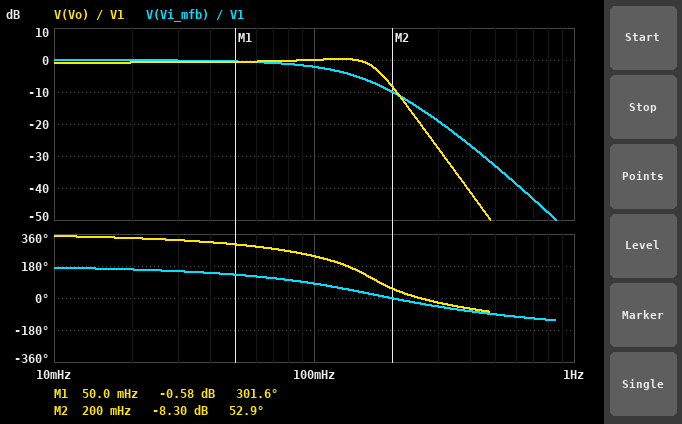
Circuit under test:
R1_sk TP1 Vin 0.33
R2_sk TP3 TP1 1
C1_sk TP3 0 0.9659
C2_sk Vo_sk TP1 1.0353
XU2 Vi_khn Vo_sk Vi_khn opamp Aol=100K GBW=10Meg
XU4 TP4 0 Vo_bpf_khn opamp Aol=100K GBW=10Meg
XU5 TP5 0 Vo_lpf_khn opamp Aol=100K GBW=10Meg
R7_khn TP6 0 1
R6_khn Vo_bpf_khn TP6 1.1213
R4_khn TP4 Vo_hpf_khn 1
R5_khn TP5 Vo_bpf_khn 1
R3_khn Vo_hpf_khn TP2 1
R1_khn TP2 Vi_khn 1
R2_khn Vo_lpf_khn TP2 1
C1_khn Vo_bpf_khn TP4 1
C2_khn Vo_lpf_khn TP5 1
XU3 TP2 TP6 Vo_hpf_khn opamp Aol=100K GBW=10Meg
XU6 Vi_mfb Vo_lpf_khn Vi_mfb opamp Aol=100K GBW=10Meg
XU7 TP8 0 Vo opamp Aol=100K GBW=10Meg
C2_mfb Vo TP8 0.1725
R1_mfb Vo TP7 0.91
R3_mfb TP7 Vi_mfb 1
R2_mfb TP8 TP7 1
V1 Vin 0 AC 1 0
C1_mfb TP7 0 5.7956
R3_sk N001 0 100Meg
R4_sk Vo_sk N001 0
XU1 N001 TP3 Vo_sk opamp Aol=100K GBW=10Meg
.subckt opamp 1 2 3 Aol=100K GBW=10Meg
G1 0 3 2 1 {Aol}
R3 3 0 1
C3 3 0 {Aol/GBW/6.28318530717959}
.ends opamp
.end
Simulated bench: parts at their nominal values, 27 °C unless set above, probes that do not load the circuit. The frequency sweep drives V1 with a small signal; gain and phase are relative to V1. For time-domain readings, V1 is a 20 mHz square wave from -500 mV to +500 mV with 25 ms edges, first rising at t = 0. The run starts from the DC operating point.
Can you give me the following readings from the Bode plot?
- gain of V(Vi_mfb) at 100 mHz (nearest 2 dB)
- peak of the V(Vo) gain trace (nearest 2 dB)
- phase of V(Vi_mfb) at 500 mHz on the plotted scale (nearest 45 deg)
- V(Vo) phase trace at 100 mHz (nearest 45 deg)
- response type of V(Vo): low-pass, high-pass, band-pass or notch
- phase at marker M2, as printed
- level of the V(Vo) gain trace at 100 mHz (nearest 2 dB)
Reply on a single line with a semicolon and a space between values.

-2 dB; 0 dB; -90 deg; 225 deg; low-pass; 52.9 deg; 0 dB
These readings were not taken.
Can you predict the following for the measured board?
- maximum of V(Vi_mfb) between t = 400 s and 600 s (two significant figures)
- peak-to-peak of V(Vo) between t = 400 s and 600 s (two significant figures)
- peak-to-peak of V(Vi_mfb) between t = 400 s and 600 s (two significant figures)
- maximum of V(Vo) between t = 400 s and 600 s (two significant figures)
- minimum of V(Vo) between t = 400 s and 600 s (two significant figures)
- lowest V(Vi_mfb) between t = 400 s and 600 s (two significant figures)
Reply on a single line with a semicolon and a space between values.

520 mV; 1.3 V; 1.0 V; 640 mV; -640 mV; -520 mV
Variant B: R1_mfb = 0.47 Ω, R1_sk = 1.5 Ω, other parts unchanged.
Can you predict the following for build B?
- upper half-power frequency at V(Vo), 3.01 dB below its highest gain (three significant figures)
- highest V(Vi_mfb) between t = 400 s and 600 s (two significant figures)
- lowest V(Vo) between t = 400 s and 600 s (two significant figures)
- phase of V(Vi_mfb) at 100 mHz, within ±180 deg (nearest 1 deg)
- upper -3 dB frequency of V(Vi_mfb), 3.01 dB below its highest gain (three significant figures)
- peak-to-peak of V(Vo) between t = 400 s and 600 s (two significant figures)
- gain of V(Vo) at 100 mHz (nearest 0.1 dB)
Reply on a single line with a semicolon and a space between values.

99.3 mHz; 500 mV; -240 mV; 49 deg; 80.7 mHz; 470 mV; -9.6 dB
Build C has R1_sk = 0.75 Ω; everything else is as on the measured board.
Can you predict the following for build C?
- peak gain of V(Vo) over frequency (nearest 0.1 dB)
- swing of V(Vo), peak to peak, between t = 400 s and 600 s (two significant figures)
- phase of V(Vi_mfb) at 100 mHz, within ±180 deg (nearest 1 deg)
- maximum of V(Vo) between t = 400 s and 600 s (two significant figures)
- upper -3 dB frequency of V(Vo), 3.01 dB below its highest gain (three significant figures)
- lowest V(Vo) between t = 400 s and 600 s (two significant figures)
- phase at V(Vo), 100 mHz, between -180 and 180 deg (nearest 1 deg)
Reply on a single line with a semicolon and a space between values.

-0.6 dB; 1.2 V; 68 deg; 600 mV; 168 mHz; -600 mV; -138 deg
